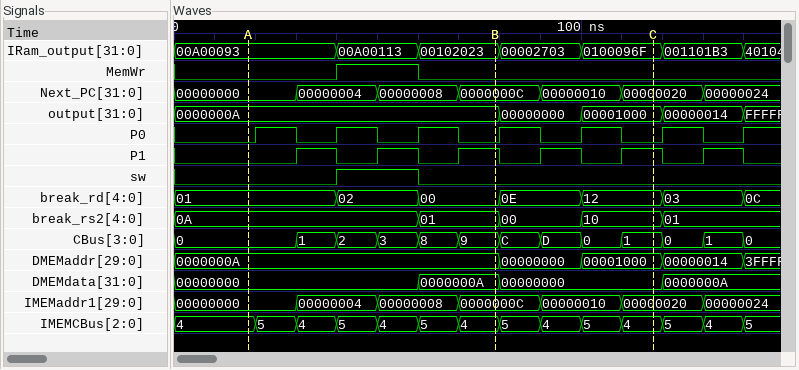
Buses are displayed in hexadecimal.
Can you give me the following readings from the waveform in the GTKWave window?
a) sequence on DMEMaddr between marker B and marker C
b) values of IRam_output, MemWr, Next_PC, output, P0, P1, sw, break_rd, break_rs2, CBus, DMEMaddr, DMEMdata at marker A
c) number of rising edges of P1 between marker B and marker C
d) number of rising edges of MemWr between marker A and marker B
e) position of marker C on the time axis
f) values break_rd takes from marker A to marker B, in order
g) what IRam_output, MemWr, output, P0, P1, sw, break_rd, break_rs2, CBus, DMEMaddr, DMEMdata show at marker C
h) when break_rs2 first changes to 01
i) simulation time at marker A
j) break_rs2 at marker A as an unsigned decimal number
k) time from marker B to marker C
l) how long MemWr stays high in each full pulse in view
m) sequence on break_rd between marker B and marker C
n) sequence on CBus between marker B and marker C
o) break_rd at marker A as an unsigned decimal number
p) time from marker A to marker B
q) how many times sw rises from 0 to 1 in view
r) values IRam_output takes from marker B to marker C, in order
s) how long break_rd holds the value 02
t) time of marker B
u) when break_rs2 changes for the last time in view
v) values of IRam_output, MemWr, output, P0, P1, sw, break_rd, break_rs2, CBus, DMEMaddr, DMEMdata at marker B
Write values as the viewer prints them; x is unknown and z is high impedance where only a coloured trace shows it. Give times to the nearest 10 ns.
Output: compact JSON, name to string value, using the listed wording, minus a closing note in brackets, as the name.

{"sequence on DMEMaddr between marker B and marker C": "0000000A, 00000000, 00001000", "values of IRam_output, MemWr, Next_PC, output, P0, P1, sw, break_rd, break_rs2, CBus, DMEMaddr, DMEMdata at marker A": "IRam_output=00A00093, MemWr=0, Next_PC=00000000, output=0000000A, P0=0, P1=0, sw=0, break_rd=01, break_rs2=0A, CBus=0, DMEMaddr=0000000A, DMEMdata=00000000", "number of rising edges of P1 between marker B and marker C": "2", "number of rising edges of MemWr between marker A and marker B": "1", "position of marker C on the time axis": "120 ns", "values break_rd takes from marker A to marker B, in order": "01, 02, 00", "what IRam_output, MemWr, output, P0, P1, sw, break_rd, break_rs2, CBus, DMEMaddr, DMEMdata show at marker C": "IRam_output=0100096F, MemWr=0, output=00001000, P0=0, P1=1, sw=0, break_rd=12, break_rs2=10, CBus=1, DMEMaddr=00001000, DMEMdata=00000000", "when break_rs2 first changes to 01": "60 ns", "simulation time at marker A": "20 ns", "break_rs2 at marker A as an unsigned decimal number": "10", "time from marker B to marker C": "40 ns", "how long MemWr stays high in each full pulse in view": "20 ns", "sequence on break_rd between marker B and marker C": "00, 0E, 12", "sequence on CBus between marker B and marker C": "9, C, D, 0, 1", "break_rd at marker A as an unsigned decimal number": "1", "time from marker A to marker B": "60 ns", "how many times sw rises from 0 to 1 in view": "1", "values IRam_output takes from marker B to marker C, in order": "00102023, 00002703, 0100096F", "how long break_rd holds the value 02": "20 ns", "time of marker B": "80 ns", "when break_rs2 changes for the last time in view": "120 ns", "values of IRam_output, MemWr, output, P0, P1, sw, break_rd, break_rs2, CBus, DMEMaddr, DMEMdata at marker B": "IRam_output=00102023, MemWr=0, output=0000000A, P0=0, P1=1, sw=0, break_rd=00, break_rs2=01, CBus=9, DMEMaddr=0000000A, DMEMdata=0000000A"}
